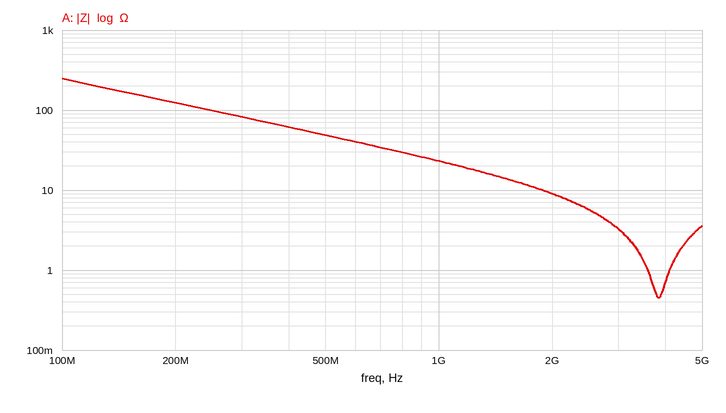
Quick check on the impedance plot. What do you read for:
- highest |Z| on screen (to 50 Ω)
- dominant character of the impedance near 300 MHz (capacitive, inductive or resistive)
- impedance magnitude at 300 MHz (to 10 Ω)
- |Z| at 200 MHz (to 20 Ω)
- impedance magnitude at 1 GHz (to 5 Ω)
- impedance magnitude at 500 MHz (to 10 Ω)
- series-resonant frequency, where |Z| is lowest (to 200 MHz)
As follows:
250 Ω
capacitive
80 Ω
120 Ω
25 Ω
50 Ω
3.8 GHz
